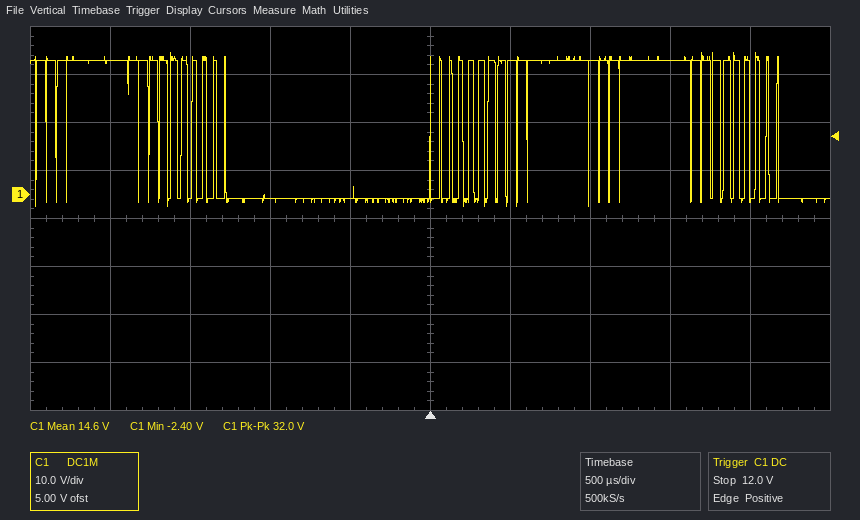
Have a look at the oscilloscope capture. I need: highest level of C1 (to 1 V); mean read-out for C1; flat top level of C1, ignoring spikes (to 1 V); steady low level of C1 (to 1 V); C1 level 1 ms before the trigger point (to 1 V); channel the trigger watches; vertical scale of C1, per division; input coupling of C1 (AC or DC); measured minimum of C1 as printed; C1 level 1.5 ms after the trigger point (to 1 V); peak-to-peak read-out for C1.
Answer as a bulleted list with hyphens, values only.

- 30 V
- 14.6 V
- 28 V
- -1 V
- -1 V
- C1
- 10 V
- DC
- -2.40 V
- 28 V
- 32.0 V
